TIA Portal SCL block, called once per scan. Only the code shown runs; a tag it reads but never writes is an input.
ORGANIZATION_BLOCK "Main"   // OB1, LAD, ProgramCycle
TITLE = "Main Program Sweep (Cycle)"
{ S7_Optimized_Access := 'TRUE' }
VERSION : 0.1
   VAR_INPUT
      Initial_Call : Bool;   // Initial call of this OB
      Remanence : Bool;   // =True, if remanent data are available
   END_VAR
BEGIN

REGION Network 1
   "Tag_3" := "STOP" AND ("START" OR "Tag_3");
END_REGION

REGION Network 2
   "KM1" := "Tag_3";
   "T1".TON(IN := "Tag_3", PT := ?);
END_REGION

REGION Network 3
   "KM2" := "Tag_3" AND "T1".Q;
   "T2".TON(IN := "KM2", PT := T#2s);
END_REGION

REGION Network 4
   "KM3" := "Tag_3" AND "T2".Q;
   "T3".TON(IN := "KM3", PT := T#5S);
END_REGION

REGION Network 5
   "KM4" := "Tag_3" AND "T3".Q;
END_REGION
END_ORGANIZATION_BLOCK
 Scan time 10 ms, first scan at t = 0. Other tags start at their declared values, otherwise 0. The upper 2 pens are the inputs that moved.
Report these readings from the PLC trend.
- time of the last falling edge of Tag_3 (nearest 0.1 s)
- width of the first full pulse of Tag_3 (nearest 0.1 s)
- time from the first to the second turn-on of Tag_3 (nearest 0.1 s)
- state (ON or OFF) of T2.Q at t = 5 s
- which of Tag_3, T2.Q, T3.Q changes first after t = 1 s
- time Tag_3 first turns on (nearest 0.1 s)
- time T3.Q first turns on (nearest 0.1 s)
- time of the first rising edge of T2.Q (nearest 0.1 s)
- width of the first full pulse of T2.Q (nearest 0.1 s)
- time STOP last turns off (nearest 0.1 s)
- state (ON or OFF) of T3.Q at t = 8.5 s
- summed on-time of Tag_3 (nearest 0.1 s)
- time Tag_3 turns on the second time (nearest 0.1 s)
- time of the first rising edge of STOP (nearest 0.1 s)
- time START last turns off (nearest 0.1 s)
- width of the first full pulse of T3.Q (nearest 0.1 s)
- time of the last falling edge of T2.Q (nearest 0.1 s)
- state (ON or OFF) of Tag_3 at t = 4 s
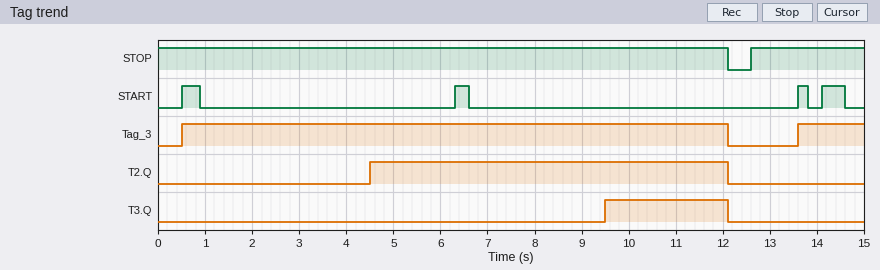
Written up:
12.1 s
11.6 s
13.1 s
ON
T2.Q
0.5 s
9.5 s
4.5 s
7.6 s
12.1 s
OFF
13.0 s
13.6 s
12.6 s
14.6 s
2.6 s
12.1 s
ON
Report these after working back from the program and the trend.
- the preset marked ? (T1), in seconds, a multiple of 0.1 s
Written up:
2.0 s
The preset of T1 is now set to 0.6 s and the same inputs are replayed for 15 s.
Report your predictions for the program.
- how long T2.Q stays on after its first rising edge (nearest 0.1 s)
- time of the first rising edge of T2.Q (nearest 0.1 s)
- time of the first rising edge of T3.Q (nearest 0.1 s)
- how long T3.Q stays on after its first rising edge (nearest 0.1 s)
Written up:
9.0 s
3.1 s
8.1 s
4.0 s
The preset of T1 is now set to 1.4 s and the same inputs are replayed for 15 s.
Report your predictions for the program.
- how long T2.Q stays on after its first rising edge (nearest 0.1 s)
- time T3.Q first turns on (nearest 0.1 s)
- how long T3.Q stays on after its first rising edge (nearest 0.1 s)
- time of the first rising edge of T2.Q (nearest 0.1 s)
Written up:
8.2 s
8.9 s
3.2 s
3.9 s
